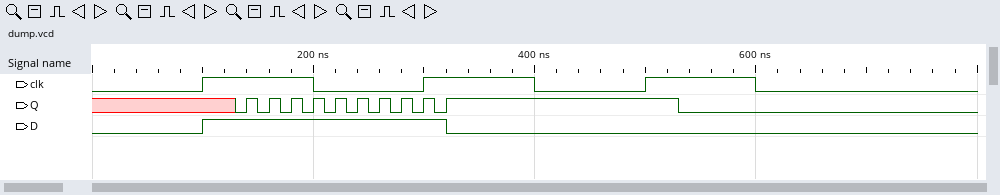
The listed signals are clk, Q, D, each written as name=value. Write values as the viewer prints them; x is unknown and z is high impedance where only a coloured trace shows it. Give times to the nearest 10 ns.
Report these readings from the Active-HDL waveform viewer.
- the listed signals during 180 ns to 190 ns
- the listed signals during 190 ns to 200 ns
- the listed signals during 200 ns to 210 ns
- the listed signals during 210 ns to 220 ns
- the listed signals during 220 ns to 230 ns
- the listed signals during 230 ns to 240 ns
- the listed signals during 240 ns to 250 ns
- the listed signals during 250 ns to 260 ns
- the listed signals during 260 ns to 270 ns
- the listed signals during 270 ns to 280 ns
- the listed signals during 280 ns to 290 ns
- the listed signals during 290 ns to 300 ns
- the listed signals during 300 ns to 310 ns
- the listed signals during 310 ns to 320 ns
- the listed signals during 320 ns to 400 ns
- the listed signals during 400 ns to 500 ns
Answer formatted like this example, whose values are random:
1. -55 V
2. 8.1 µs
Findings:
1. clk=1, Q=1, D=1
2. clk=1, Q=0, D=1
3. clk=0, Q=1, D=1
4. clk=0, Q=0, D=1
5. clk=0, Q=1, D=1
6. clk=0, Q=0, D=1
7. clk=0, Q=1, D=1
8. clk=0, Q=0, D=1
9. clk=0, Q=1, D=1
10. clk=0, Q=0, D=1
11. clk=0, Q=1, D=1
12. clk=0, Q=0, D=1
13. clk=1, Q=1, D=1
14. clk=1, Q=0, D=1
15. clk=1, Q=1, D=0
16. clk=0, Q=1, D=0
